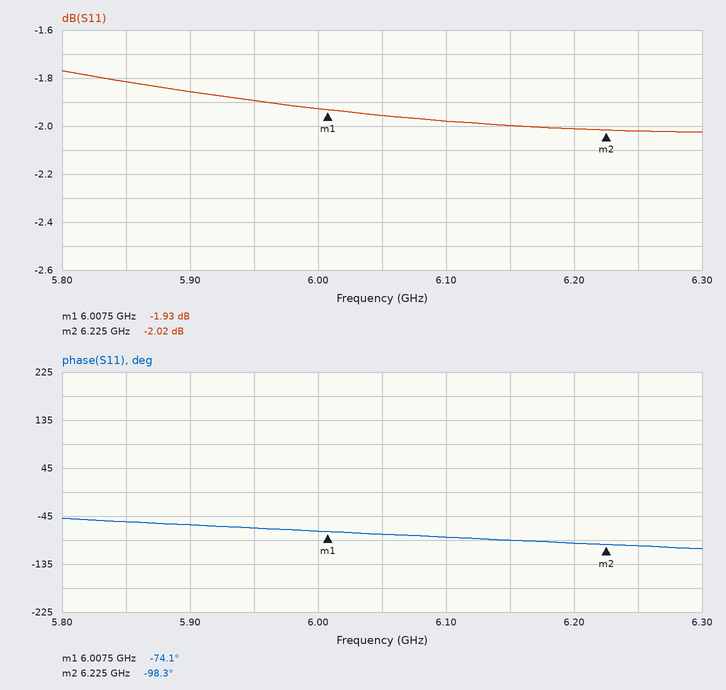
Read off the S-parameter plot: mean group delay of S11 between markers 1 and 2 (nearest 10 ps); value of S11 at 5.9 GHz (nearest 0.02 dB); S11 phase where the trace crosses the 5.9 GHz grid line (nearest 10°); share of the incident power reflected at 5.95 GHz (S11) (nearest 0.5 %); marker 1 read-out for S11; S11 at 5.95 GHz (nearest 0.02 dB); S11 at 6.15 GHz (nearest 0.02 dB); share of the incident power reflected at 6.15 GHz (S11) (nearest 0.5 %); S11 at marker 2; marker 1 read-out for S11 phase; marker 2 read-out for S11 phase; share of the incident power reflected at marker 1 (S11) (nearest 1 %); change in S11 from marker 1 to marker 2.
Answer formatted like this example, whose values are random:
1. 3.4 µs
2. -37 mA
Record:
1. 310 ps
2. -1.86 dB
3. -60°
4. 64.5 %
5. -1.93 dB
6. -1.90 dB
7. -2.00 dB
8. 63.0 %
9. -2.02 dB
10. -74.1°
11. -98.3°
12. 64 %
13. -0.09 dB
